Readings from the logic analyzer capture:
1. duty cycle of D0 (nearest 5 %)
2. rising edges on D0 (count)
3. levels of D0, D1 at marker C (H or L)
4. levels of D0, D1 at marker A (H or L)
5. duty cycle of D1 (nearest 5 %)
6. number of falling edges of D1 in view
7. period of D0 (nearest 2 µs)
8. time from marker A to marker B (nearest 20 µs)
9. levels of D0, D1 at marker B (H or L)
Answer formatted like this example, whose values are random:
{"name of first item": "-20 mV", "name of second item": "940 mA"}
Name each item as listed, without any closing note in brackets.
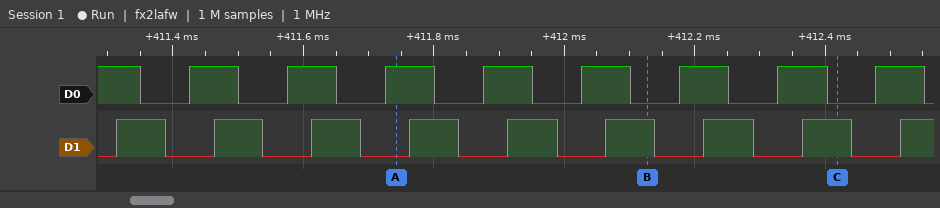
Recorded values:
{"duty cycle of D0": "50 %", "rising edges on D0": "8", "levels of D0, D1 at marker C": "D0=L, D1=H", "levels of D0, D1 at marker A": "D0=H, D1=L", "duty cycle of D1": "50 %", "number of falling edges of D1 in view": "8", "period of D0": "150 µs", "time from marker A to marker B": "380 µs", "levels of D0, D1 at marker B": "D0=L, D1=H"}
